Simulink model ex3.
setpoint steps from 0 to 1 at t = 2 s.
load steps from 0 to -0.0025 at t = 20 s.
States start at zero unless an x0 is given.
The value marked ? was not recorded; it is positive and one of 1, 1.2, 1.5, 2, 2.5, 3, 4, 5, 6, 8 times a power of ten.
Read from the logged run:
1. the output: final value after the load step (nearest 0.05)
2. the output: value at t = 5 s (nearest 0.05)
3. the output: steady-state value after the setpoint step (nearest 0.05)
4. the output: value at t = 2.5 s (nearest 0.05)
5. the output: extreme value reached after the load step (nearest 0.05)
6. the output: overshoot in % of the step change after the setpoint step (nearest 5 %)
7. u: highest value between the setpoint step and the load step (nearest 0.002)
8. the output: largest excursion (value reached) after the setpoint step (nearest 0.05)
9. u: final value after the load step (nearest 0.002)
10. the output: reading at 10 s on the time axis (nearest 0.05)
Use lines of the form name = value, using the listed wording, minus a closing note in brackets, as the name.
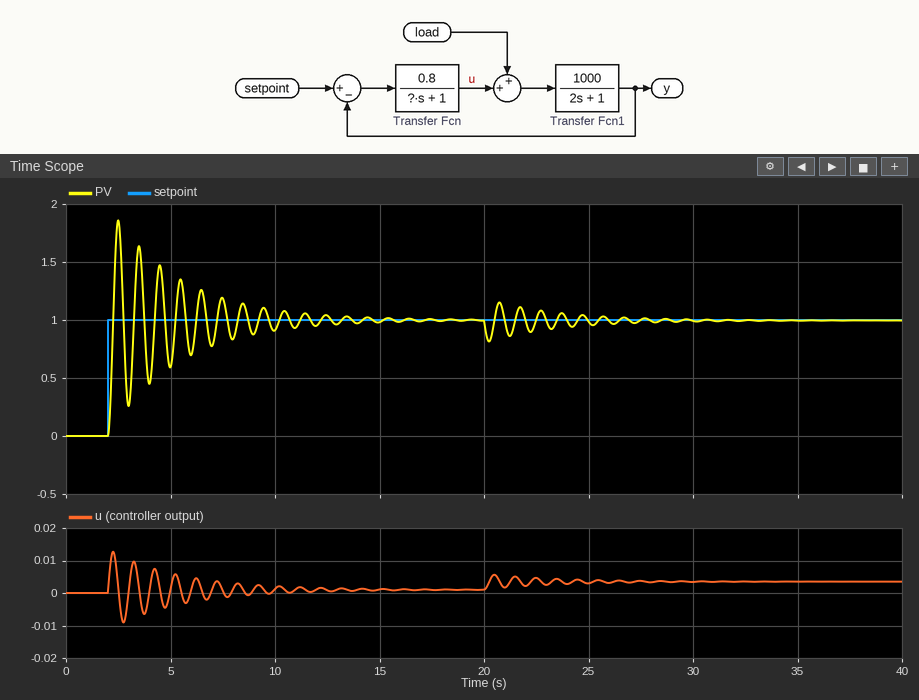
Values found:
the output: final value after the load step = 1.00
the output: value at t = 5 s = 0.60
the output: steady-state value after the setpoint step = 1.00
the output: value at t = 2.5 s = 1.85
the output: extreme value reached after the load step = 0.80
the output: overshoot in % of the step change after the setpoint step = 85 %
u: highest value between the setpoint step and the load step = 0.012
the output: largest excursion (value reached) after the setpoint step = 1.85
u: final value after the load step = 0.004
the output: reading at 10 s on the time axis = 0.90
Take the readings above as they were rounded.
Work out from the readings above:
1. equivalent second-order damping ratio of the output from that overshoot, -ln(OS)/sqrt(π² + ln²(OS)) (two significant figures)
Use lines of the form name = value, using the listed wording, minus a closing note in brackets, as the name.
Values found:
equivalent second-order damping ratio of the output from that overshoot, -ln(OS)/sqrt(π² + ln²(OS)) = 0.052
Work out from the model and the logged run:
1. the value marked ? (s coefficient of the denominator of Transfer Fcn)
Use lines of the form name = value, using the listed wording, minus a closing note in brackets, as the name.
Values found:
the value marked ? = 10
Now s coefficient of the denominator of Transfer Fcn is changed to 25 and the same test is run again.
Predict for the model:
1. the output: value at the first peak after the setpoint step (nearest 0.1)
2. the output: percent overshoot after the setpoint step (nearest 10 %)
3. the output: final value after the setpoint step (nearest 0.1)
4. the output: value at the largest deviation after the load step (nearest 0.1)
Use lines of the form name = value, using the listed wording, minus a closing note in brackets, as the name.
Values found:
the output: value at the first peak after the setpoint step = 1.8
the output: percent overshoot after the setpoint step = 80 %
the output: final value after the setpoint step = 1.0
the output: value at the largest deviation after the load step = 0.7
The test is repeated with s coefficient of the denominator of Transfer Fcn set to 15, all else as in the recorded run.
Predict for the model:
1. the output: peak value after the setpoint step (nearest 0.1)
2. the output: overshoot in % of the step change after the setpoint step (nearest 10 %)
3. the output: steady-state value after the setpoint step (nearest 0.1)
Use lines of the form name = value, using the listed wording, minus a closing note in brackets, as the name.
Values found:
the output: peak value after the setpoint step = 1.8
the output: overshoot in % of the step change after the setpoint step = 80 %
the output: steady-state value after the setpoint step = 1.0
